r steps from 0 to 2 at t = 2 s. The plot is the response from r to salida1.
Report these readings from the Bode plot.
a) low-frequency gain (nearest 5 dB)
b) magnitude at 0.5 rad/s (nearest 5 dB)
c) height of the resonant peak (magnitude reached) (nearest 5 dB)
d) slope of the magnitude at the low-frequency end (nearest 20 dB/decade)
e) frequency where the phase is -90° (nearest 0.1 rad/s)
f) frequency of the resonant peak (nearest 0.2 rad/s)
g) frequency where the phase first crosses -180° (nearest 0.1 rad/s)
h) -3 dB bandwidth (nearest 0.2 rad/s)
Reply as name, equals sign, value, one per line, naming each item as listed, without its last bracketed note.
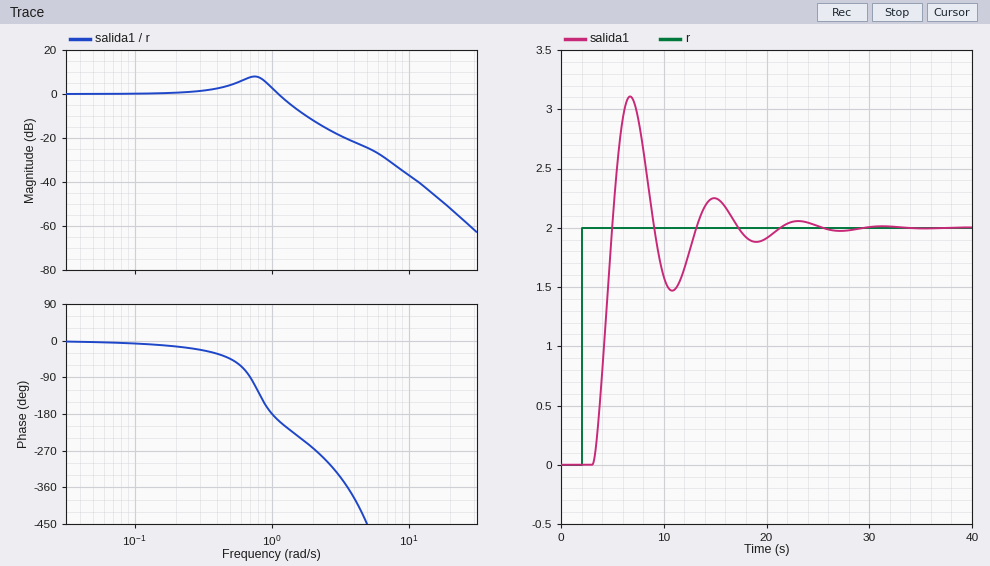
low-frequency gain = 0 dB
magnitude at 0.5 rad/s = 5 dB
height of the resonant peak (magnitude reached) = 10 dB
slope of the magnitude at the low-frequency end = 0 dB/decade
frequency where the phase is -90° = 0.7 rad/s
frequency of the resonant peak = 0.8 rad/s
frequency where the phase first crosses -180° = 1.0 rad/s
-3 dB bandwidth = 1.2 rad/s
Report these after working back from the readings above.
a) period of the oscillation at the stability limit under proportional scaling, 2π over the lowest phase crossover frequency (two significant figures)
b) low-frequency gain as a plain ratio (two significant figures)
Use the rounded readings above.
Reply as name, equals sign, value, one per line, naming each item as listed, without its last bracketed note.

period of the oscillation at the stability limit under proportional scaling, 2π over the lowest phase crossover frequency = 6.3 s
low-frequency gain as a plain ratio = 1.0
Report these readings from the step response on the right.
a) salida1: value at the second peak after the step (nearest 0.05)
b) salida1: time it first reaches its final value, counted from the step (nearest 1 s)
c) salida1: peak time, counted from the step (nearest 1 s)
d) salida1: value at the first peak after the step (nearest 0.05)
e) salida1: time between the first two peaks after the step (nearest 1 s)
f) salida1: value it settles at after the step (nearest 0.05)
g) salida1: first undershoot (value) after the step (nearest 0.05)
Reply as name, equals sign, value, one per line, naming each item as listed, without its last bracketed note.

salida1: value at the second peak after the step = 2.25
salida1: time it first reaches its final value, counted from the step = 3 s
salida1: peak time, counted from the step = 5 s
salida1: value at the first peak after the step = 3.10
salida1: time between the first two peaks after the step = 8 s
salida1: value it settles at after the step = 2.00
salida1: first undershoot (value) after the step = 1.45
